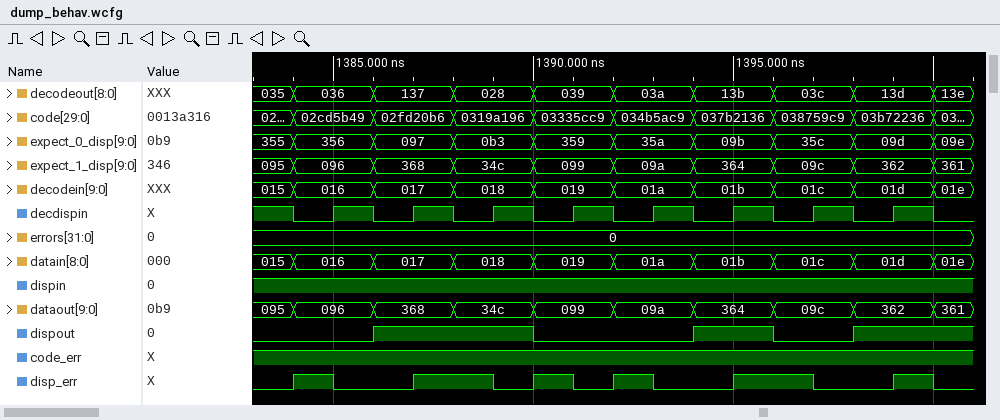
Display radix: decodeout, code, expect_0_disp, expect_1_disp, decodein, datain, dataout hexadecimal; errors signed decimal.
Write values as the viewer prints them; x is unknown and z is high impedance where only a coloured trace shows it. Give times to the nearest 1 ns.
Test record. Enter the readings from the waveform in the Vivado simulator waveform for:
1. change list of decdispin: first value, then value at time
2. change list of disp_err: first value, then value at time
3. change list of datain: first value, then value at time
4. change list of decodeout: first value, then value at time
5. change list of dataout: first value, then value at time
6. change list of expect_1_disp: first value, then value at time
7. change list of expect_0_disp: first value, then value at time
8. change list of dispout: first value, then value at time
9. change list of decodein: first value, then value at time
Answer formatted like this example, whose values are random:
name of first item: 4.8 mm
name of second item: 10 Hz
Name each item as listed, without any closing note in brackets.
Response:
change list of decdispin: first value, then value at time: 1, 0 at 1384 ns, 1 at 1385 ns, 0 at 1386 ns, 1 at 1387 ns, 0 at 1388 ns, 1 at 1389 ns, 0 at 1390 ns, 1 at 1391 ns, 0 at 1392 ns, 1 at 1393 ns, 0 at 1394 ns, 1 at 1395 ns, 0 at 1396 ns, 1 at 1397 ns, 0 at 1398 ns, 1 at 1399 ns, 0 at 1400 ns
change list of disp_err: first value, then value at time: 0, 1 at 1384 ns, 0 at 1385 ns, 1 at 1387 ns, 0 at 1389 ns, 1 at 1390 ns, 0 at 1391 ns, 1 at 1392 ns, 0 at 1393 ns, 1 at 1395 ns, 0 at 1397 ns, 1 at 1399 ns, 0 at 1400 ns
change list of datain: first value, then value at time: 015, 016 at 1384 ns, 017 at 1386 ns, 018 at 1388 ns, 019 at 1390 ns, 01a at 1392 ns, 01b at 1394 ns, 01c at 1396 ns, 01d at 1398 ns, 01e at 1400 ns
change list of decodeout: first value, then value at time: 035, 036 at 1384 ns, 137 at 1386 ns, 028 at 1388 ns, 039 at 1390 ns, 03a at 1392 ns, 13b at 1394 ns, 03c at 1396 ns, 13d at 1398 ns, 13e at 1400 ns
change list of dataout: first value, then value at time: 095, 096 at 1384 ns, 368 at 1386 ns, 34c at 1388 ns, 099 at 1390 ns, 09a at 1392 ns, 364 at 1394 ns, 09c at 1396 ns, 362 at 1398 ns, 361 at 1400 ns
change list of expect_1_disp: first value, then value at time: 095, 096 at 1384 ns, 368 at 1386 ns, 34c at 1388 ns, 099 at 1390 ns, 09a at 1392 ns, 364 at 1394 ns, 09c at 1396 ns, 362 at 1398 ns, 361 at 1400 ns
change list of expect_0_disp: first value, then value at time: 355, 356 at 1384 ns, 097 at 1386 ns, 0b3 at 1388 ns, 359 at 1390 ns, 35a at 1392 ns, 09b at 1394 ns, 35c at 1396 ns, 09d at 1398 ns, 09e at 1400 ns
change list of dispout: first value, then value at time: 0, 1 at 1386 ns, 0 at 1390 ns, 1 at 1394 ns, 0 at 1396 ns, 1 at 1398 ns
change list of decodein: first value, then value at time: 015, 016 at 1384 ns, 017 at 1386 ns, 018 at 1388 ns, 019 at 1390 ns, 01a at 1392 ns, 01b at 1394 ns, 01c at 1396 ns, 01d at 1398 ns, 01e at 1400 ns
